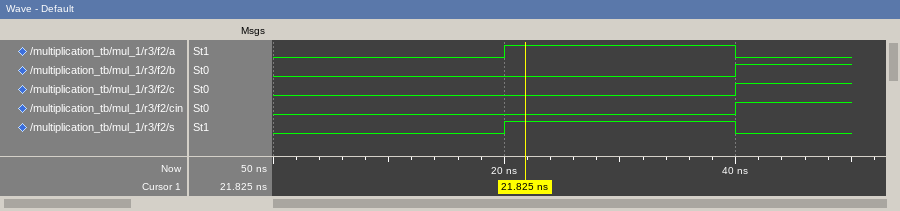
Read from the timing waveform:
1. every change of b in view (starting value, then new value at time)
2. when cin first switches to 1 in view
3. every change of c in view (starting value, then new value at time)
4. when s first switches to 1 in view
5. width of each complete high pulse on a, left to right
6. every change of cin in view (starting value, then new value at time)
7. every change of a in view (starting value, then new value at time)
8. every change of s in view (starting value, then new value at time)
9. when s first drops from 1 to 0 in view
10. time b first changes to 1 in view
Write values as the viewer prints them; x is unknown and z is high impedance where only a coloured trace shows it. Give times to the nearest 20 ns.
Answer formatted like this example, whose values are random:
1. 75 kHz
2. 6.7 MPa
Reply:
1. 0, 1 at 40 ns
2. 40 ns
3. 0, 1 at 40 ns
4. 20 ns
5. 20 ns
6. 0, 1 at 40 ns
7. 0, 1 at 20 ns, 0 at 40 ns
8. 0, 1 at 20 ns, 0 at 40 ns
9. 40 ns
10. 40 ns
